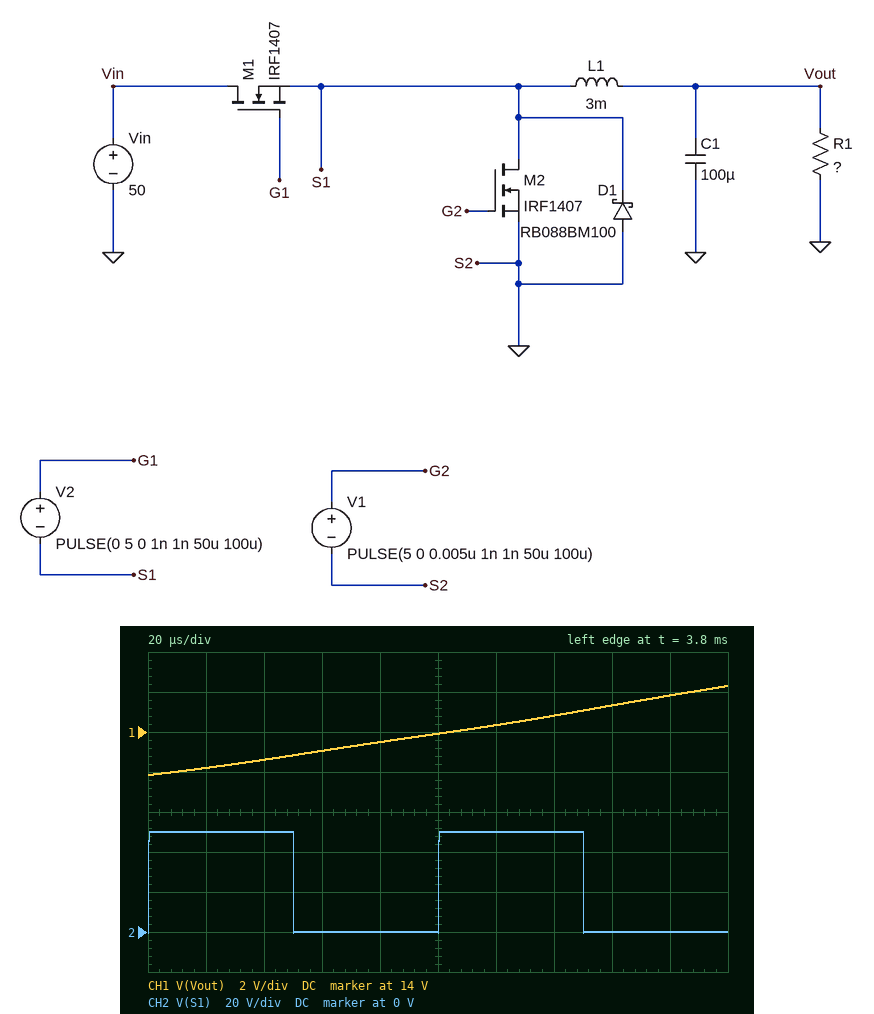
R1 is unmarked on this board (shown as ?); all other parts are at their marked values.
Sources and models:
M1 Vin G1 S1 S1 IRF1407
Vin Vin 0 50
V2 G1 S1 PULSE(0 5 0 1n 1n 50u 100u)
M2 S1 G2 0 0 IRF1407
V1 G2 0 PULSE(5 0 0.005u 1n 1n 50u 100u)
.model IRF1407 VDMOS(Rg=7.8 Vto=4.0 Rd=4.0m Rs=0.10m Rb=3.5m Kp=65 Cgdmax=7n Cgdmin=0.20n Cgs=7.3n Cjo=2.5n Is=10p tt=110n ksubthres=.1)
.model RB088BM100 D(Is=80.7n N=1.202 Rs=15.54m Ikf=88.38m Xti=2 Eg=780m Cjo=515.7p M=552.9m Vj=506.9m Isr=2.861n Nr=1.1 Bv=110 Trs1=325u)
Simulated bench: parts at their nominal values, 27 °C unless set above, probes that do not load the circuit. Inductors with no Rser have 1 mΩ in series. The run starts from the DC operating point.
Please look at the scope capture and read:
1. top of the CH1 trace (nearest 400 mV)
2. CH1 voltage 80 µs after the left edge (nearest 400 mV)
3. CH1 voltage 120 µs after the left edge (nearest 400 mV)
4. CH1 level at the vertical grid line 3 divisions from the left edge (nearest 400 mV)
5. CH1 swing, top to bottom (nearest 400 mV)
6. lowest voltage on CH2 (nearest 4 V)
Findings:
16.4 V
13.6 V
14.4 V
13.2 V
4.4 V
0 V
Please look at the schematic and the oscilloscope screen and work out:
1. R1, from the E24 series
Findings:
47 Ω
